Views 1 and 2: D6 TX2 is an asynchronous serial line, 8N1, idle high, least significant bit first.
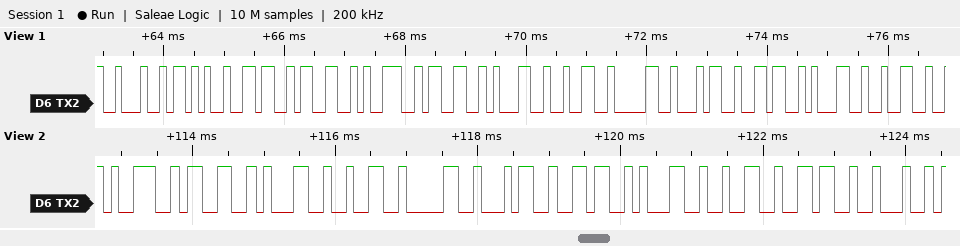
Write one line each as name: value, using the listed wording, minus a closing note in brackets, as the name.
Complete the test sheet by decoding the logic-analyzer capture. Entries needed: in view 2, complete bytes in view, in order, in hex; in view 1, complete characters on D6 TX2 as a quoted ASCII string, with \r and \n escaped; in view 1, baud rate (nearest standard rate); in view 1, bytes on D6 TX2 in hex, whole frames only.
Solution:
in view 2, complete bytes in view, in order, in hex: 0x39 0x33 0x31 0x32 0x30 0x34 0x36 0x31 0x32 0x36 0x22
in view 1, complete characters on D6 TX2 as a quoted ASCII string, with \r and \n escaped: "\"+63931204612"
in view 1, baud rate: 9600 baud
in view 1, bytes on D6 TX2 in hex, whole frames only: 22 2B 36 33 39 33 31 32 30 34 36 31 32
